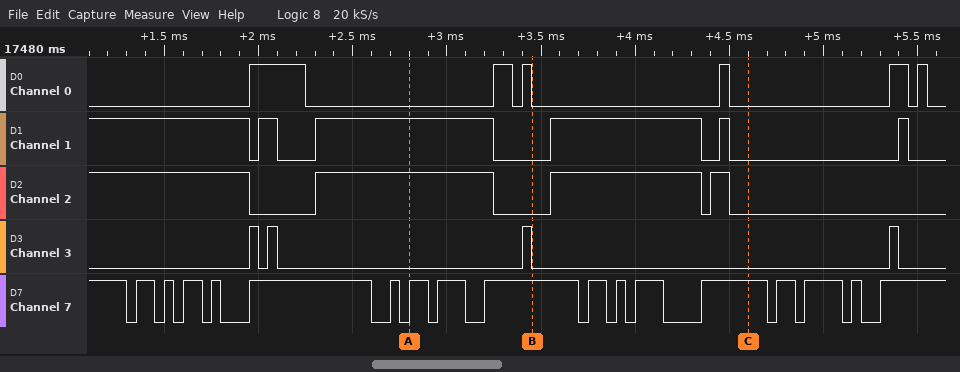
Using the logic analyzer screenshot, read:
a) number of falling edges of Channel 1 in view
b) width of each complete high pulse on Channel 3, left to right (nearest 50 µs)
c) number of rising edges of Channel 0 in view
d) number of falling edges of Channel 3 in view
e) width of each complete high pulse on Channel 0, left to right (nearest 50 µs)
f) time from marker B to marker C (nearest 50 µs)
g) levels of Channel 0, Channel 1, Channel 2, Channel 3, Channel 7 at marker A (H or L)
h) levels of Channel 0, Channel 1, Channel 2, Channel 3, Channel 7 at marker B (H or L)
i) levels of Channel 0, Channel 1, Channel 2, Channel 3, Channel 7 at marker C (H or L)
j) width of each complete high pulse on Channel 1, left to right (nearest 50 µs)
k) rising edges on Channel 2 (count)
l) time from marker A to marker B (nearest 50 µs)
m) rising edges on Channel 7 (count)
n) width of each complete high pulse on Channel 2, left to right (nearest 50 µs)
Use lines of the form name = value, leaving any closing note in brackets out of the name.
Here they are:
number of falling edges of Channel 1 in view = 6
width of each complete high pulse on Channel 3, left to right = 50 µs, 50 µs, 50 µs, 50 µs
number of rising edges of Channel 0 in view = 6
number of falling edges of Channel 3 in view = 4
width of each complete high pulse on Channel 0, left to right = 300 µs, 100 µs, 50 µs, 50 µs, 100 µs, 50 µs
time from marker B to marker C = 1150 µs
levels of Channel 0, Channel 1, Channel 2, Channel 3, Channel 7 at marker A = Channel 0=L, Channel 1=H, Channel 2=H, Channel 3=L, Channel 7=H
levels of Channel 0, Channel 1, Channel 2, Channel 3, Channel 7 at marker B = Channel 0=L, Channel 1=L, Channel 2=L, Channel 3=L, Channel 7=H
levels of Channel 0, Channel 1, Channel 2, Channel 3, Channel 7 at marker C = Channel 0=L, Channel 1=L, Channel 2=L, Channel 3=L, Channel 7=H
width of each complete high pulse on Channel 1, left to right = 100 µs, 950 µs, 800 µs, 50 µs, 50 µs
rising edges on Channel 2 = 3
time from marker A to marker B = 650 µs
rising edges on Channel 7 = 17
width of each complete high pulse on Channel 2, left to right = 950 µs, 800 µs, 100 µs
